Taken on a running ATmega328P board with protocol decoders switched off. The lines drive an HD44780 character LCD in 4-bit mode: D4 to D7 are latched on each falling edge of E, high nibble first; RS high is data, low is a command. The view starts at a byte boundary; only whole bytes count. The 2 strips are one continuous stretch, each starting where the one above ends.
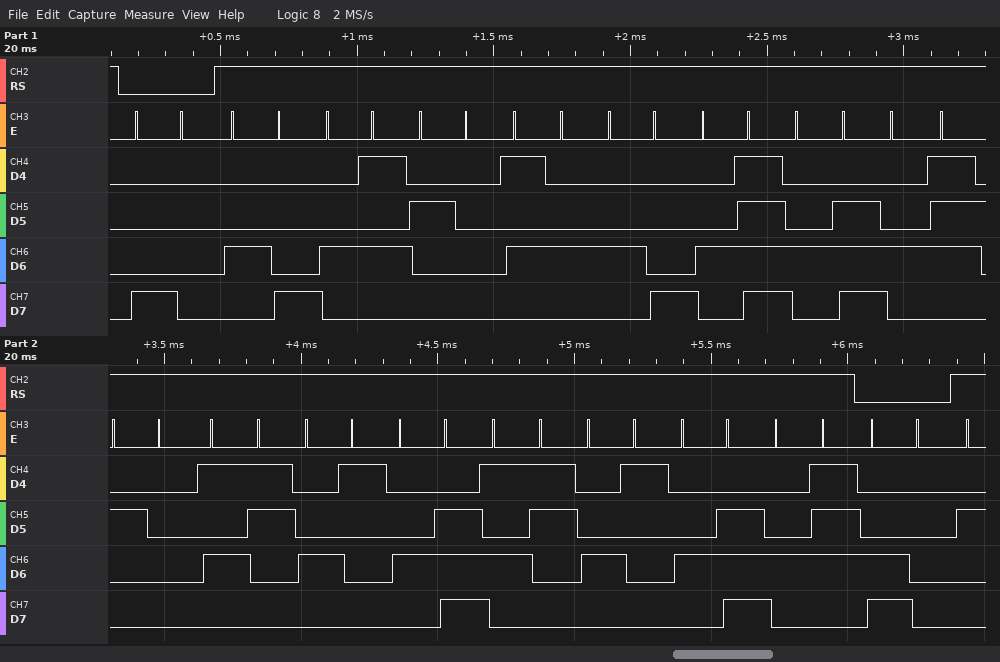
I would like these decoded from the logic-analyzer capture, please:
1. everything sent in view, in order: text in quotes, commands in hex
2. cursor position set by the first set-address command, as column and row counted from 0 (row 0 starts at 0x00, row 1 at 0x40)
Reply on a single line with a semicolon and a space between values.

0x80 "HE THONG SANSANG" 0xC0; column 0, row 0
